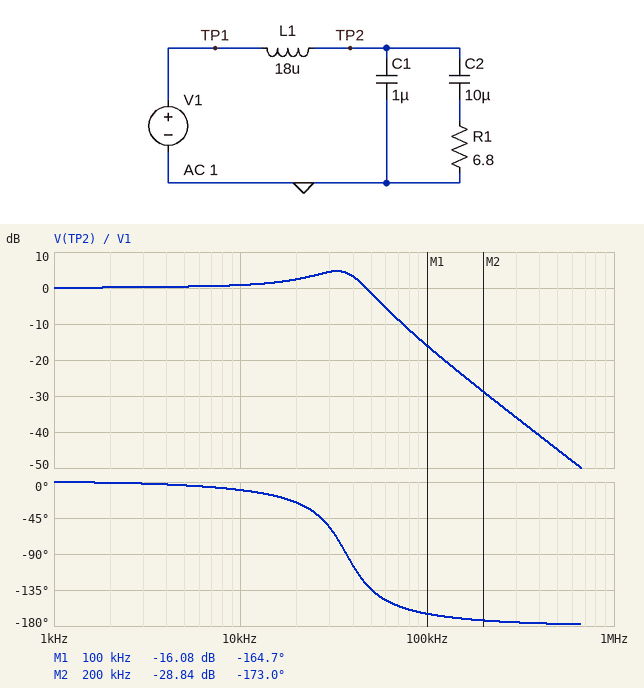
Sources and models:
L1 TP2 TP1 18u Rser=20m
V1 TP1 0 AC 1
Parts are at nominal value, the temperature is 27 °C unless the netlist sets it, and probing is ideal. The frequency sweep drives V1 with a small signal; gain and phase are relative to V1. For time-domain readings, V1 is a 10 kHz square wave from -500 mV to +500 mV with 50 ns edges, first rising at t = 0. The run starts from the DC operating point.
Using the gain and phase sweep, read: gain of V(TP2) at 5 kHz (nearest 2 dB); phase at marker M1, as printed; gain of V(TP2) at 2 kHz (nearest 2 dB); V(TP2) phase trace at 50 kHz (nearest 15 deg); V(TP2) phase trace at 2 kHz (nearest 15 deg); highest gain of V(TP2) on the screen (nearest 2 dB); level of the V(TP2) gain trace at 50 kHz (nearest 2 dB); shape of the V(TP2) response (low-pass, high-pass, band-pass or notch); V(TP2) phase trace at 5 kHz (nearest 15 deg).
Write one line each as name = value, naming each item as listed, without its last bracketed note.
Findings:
gain of V(TP2) at 5 kHz = 0 dB
phase at marker M1, as printed = -164.7 deg
gain of V(TP2) at 2 kHz = 0 dB
V(TP2) phase trace at 50 kHz = -135 deg
V(TP2) phase trace at 2 kHz = 0 deg
highest gain of V(TP2) on the screen = 4 dB
level of the V(TP2) gain trace at 50 kHz = -2 dB
shape of the V(TP2) response = low-pass
V(TP2) phase trace at 5 kHz = 0 deg
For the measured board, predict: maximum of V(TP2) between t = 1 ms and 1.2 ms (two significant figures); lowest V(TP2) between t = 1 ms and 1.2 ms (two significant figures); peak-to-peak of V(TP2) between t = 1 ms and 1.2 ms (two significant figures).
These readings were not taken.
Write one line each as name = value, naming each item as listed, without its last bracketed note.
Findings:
maximum of V(TP2) between t = 1 ms and 1.2 ms = 890 mV
lowest V(TP2) between t = 1 ms and 1.2 ms = -890 mV
peak-to-peak of V(TP2) between t = 1 ms and 1.2 ms = 1.8 V
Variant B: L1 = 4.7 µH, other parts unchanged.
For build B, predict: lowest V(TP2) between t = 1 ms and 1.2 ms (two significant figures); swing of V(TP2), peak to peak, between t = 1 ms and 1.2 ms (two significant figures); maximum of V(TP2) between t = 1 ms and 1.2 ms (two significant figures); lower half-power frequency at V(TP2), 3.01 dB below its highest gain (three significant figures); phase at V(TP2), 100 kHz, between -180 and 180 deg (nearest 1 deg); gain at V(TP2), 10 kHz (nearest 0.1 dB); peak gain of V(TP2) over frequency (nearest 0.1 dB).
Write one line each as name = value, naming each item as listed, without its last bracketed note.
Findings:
lowest V(TP2) between t = 1 ms and 1.2 ms = -1.1 V
swing of V(TP2), peak to peak, between t = 1 ms and 1.2 ms = 2.2 V
maximum of V(TP2) between t = 1 ms and 1.2 ms = 1.1 V
lower half-power frequency at V(TP2), 3.01 dB below its highest gain = 57.7 kHz
phase at V(TP2), 100 kHz, between -180 and 180 deg = -153 deg
gain at V(TP2), 10 kHz = 0.2 dB
peak gain of V(TP2) over frequency = 9.8 dB
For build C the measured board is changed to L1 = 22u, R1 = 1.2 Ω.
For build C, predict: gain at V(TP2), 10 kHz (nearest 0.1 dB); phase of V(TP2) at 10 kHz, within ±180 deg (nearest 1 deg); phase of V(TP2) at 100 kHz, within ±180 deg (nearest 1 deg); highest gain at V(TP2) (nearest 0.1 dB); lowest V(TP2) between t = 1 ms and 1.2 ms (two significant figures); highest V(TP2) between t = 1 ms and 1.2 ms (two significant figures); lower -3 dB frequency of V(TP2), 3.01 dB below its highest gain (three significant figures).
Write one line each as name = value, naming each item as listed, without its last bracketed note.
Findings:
gain at V(TP2), 10 kHz = 5.0 dB
phase of V(TP2) at 10 kHz, within ±180 deg = -49 deg
phase of V(TP2) at 100 kHz, within ±180 deg = -129 deg
highest gain at V(TP2) = 5.1 dB
lowest V(TP2) between t = 1 ms and 1.2 ms = -1.1 V
highest V(TP2) between t = 1 ms and 1.2 ms = 1.1 V
lower -3 dB frequency of V(TP2), 3.01 dB below its highest gain = 5.06 kHz
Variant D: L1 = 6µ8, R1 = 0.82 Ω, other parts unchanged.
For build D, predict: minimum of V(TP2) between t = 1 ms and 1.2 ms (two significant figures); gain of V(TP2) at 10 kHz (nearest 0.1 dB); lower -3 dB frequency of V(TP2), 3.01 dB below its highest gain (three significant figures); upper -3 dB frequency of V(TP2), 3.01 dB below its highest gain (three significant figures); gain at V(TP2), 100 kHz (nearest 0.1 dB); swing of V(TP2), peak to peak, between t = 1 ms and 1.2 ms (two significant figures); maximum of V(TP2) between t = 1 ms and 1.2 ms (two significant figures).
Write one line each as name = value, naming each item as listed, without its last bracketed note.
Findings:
minimum of V(TP2) between t = 1 ms and 1.2 ms = -840 mV
gain of V(TP2) at 10 kHz = 2.2 dB
lower -3 dB frequency of V(TP2), 3.01 dB below its highest gain = 6.25 kHz
upper -3 dB frequency of V(TP2), 3.01 dB below its highest gain = 25.9 kHz
gain at V(TP2), 100 kHz = -15.1 dB
swing of V(TP2), peak to peak, between t = 1 ms and 1.2 ms = 1.7 V
maximum of V(TP2) between t = 1 ms and 1.2 ms = 840 mV
